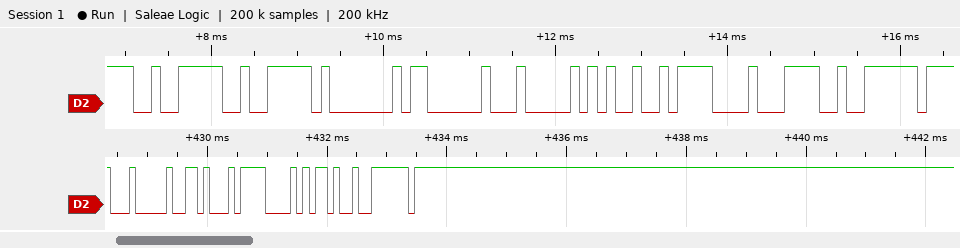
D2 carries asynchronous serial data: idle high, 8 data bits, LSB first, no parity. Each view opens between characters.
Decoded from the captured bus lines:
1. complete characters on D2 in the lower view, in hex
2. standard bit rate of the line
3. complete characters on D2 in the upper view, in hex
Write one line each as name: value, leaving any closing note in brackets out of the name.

complete characters on D2 in the lower view, in hex: 04, 16, 0F, 2D, 7E
standard bit rate of the line: 9600 baud
complete characters on D2 in the upper view, in hex: F2, F2, 01, 03, 04, 25, 0F, 3C, 7E
